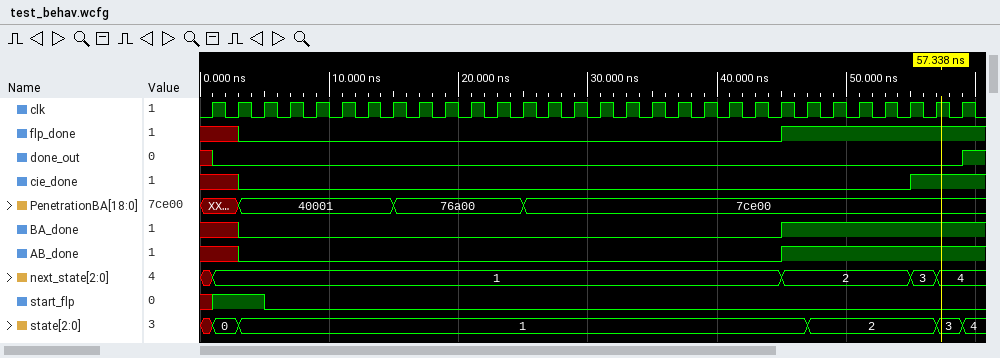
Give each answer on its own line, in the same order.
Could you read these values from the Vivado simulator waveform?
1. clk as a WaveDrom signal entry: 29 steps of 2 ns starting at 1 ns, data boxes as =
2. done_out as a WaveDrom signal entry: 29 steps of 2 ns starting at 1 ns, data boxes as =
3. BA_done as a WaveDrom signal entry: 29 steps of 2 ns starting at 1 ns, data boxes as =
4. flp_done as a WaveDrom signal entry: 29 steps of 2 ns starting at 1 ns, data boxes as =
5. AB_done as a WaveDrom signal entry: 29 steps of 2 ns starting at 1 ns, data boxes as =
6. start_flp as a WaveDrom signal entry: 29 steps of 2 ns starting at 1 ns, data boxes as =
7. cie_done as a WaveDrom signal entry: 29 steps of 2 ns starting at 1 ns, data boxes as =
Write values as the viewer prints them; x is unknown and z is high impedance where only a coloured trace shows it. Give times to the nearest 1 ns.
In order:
{name: 'clk', wave: 'p............................'}
{name: 'done_out', wave: '0............................'}
{name: 'BA_done', wave: 'x0....................1......'}
{name: 'flp_done', wave: 'x0....................1......'}
{name: 'AB_done', wave: 'x0....................1......'}
{name: 'start_flp', wave: '1.0..........................'}
{name: 'cie_done', wave: 'x0.........................1.'}
